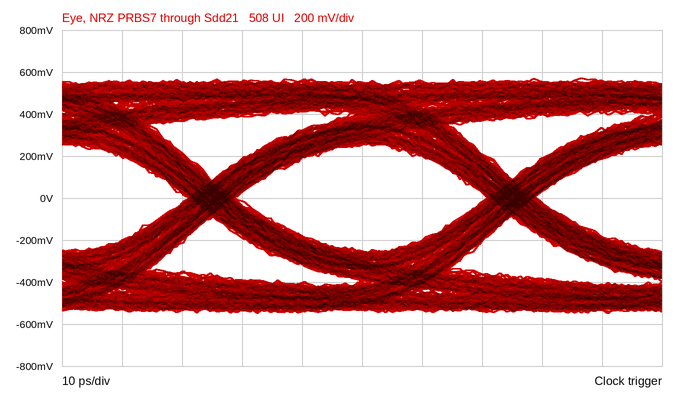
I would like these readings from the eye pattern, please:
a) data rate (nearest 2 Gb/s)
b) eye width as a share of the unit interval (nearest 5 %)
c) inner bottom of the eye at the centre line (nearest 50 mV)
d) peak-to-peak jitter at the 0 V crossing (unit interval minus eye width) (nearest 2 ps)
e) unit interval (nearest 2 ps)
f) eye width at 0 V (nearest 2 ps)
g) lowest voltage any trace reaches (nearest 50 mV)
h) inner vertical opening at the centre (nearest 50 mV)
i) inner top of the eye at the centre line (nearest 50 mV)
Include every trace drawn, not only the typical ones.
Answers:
20 Gb/s
85 %
-250 mV
8 ps
50 ps
42 ps
-550 mV
500 mV
250 mV
